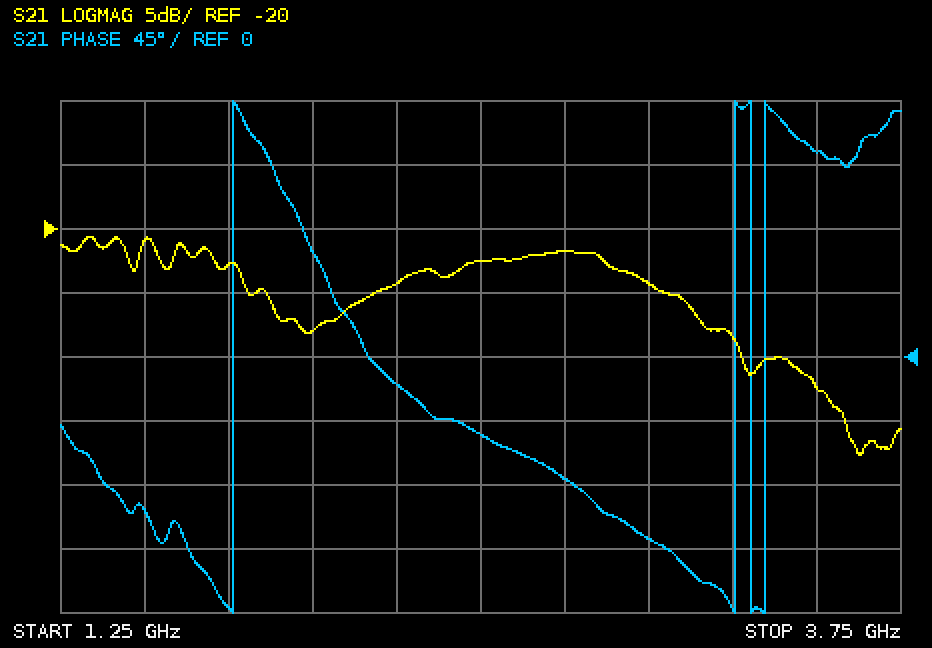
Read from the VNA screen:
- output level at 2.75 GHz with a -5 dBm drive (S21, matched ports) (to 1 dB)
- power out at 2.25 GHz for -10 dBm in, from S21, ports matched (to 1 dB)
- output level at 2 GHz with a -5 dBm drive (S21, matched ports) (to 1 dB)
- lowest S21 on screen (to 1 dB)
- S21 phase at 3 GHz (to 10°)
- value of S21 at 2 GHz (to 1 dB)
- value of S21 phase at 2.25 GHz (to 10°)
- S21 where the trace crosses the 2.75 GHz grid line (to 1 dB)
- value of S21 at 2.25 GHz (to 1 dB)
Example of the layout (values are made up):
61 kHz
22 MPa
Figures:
-27 dBm
-34 dBm
-33 dBm
-38 dB
-130°
-28 dB
-20°
-22 dB
-24 dB
